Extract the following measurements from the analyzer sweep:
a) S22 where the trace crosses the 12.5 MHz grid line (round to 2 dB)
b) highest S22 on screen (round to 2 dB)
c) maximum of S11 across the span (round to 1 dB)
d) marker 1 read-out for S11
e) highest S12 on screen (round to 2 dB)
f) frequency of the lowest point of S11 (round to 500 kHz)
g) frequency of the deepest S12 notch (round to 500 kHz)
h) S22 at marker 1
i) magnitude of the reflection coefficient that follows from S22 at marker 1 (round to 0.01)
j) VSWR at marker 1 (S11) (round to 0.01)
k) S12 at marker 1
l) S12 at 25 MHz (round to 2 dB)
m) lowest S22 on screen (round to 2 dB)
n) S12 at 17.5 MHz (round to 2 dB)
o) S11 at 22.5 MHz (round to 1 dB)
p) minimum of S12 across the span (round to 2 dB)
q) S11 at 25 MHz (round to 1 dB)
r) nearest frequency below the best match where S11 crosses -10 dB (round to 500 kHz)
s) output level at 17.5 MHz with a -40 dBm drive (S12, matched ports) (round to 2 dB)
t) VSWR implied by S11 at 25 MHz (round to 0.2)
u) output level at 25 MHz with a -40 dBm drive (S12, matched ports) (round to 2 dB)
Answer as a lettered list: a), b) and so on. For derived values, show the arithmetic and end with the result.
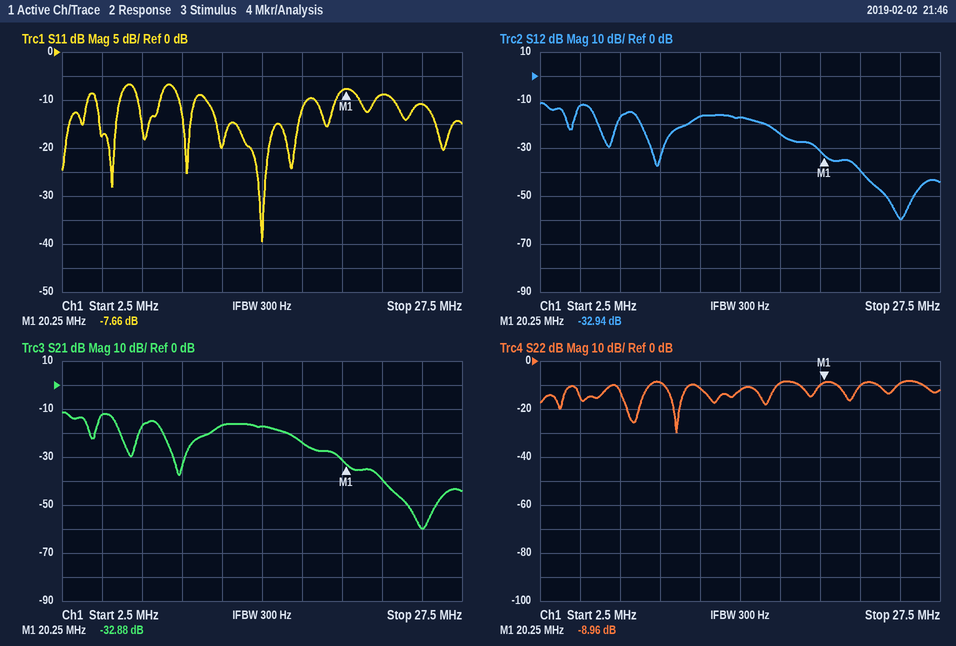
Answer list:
a) -12 dB
b) -8 dB
c) -7 dB
d) -7.66 dB
e) -12 dB
f) 15.0 MHz
g) 25.0 MHz
h) -8.96 dB
i) 10^(-8.96/20) ≈ 0.36
j) (1 + 0.4140)/(1 − 0.4140) ≈ 2.41
k) -32.94 dB
l) -60 dB
m) -30 dB
n) -24 dB
o) -9 dB
p) -60 dB
q) -11 dB
r) 11.5 MHz
s) -40 dBm + (-24 dB) = -64 dBm
t) |Γ| = 10^(-11/20) = 0.2818; VSWR = (1 + 0.2818)/(1 − 0.2818) ≈ 1.8
u) -40 dBm + (-60 dB) = -100 dBm
